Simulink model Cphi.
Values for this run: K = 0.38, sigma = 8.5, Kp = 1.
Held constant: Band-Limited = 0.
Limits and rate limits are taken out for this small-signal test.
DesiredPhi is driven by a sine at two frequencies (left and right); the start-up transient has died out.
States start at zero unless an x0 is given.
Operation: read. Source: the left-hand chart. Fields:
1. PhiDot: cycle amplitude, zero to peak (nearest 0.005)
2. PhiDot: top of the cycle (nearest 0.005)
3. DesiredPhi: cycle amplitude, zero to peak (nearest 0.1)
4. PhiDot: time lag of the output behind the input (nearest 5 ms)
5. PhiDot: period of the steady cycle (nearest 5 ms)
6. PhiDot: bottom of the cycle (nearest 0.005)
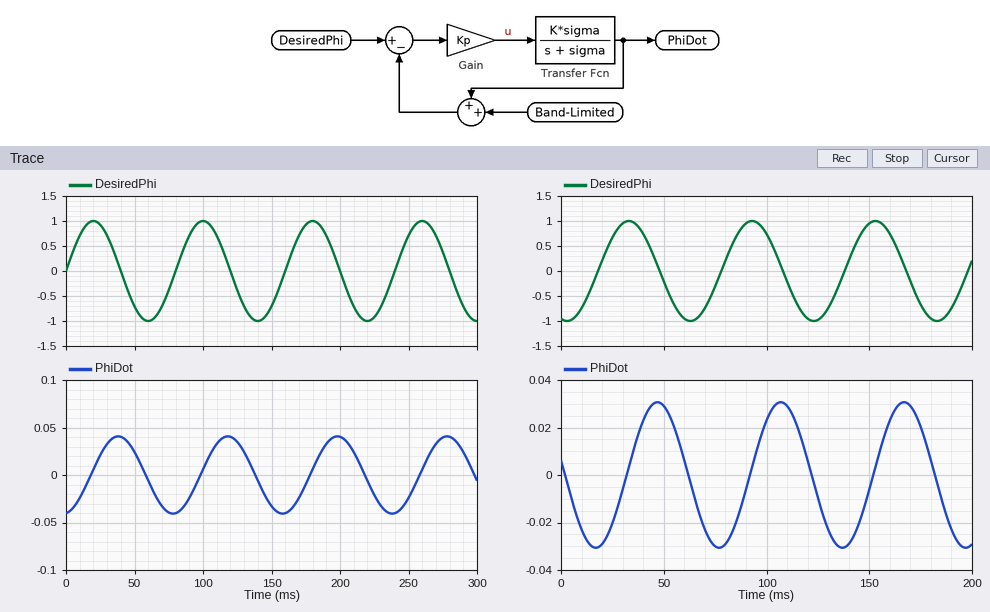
0.040
0.040
1.0
20 ms
80 ms
-0.040
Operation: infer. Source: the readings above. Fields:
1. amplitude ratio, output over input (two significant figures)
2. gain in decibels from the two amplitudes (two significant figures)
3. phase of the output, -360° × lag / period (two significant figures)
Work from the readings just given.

0.040
-28 dB
-90°
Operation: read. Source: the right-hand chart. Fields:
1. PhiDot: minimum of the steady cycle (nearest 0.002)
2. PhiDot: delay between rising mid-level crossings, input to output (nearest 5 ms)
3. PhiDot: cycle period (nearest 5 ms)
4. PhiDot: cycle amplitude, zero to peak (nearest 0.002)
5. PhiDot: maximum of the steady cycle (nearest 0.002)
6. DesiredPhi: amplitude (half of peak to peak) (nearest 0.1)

-0.030
15 ms
60 ms
0.030
0.030
1.0
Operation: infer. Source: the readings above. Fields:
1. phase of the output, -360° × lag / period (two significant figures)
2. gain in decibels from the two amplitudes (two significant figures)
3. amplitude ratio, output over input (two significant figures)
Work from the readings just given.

-90°
-30 dB
0.030
